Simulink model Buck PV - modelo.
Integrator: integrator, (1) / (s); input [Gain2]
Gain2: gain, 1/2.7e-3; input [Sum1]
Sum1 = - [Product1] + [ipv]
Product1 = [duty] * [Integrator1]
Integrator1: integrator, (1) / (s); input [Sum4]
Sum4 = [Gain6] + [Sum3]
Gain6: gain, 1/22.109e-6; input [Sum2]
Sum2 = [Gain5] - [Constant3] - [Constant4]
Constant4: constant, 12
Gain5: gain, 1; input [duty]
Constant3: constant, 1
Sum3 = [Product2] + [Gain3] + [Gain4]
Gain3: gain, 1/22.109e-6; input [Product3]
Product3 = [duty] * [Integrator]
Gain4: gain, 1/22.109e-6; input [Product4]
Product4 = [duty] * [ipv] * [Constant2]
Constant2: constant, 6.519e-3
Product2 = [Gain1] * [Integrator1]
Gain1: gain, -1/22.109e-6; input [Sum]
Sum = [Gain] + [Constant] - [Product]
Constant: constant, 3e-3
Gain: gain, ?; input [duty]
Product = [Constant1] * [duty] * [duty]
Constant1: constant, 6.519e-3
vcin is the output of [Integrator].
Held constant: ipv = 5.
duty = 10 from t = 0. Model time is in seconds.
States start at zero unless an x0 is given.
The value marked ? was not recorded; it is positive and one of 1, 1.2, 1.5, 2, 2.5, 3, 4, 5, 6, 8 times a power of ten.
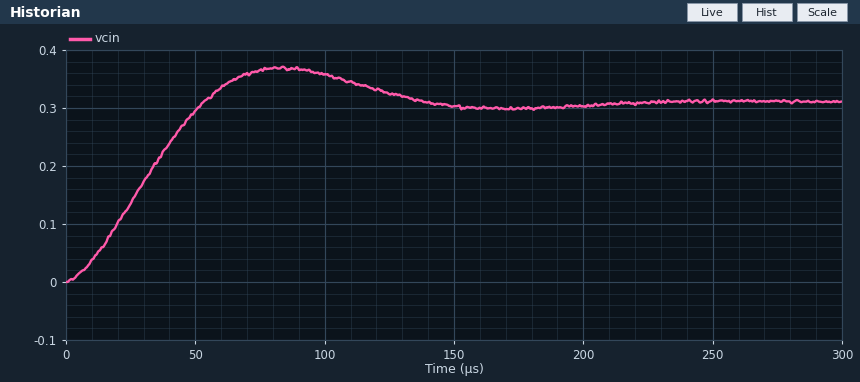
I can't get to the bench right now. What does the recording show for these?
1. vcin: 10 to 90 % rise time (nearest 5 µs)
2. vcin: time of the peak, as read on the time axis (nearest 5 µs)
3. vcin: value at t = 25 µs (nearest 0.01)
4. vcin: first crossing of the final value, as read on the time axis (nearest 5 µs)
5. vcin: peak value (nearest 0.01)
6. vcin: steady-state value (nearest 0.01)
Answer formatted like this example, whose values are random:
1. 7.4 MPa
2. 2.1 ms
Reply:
1. 40 µs
2. 85 µs
3. 0.14
4. 55 µs
5. 0.37
6. 0.31
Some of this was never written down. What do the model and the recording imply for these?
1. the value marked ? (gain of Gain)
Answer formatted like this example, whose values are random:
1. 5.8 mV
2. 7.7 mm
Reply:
1. 0.15
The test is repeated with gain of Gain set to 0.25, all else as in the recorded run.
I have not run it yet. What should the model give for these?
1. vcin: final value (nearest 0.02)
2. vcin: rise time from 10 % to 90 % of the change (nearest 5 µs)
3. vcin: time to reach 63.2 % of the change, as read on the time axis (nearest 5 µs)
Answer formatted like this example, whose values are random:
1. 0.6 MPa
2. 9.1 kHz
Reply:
1. 0.36
2. 85 µs
3. 50 µs
